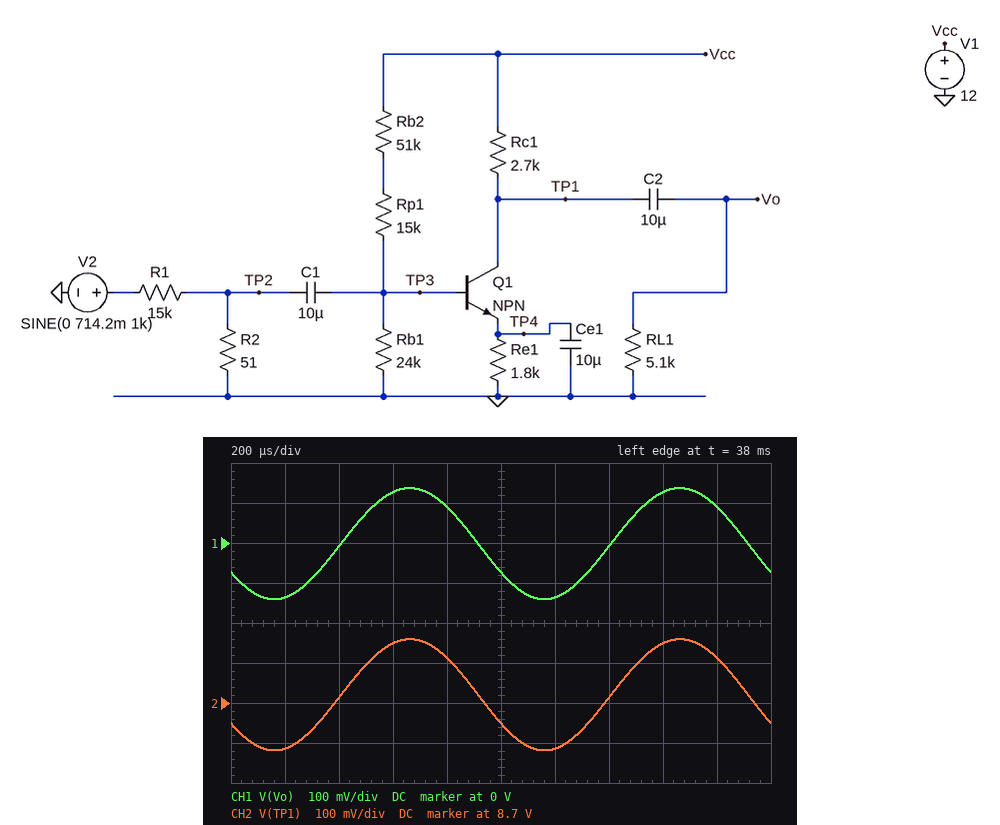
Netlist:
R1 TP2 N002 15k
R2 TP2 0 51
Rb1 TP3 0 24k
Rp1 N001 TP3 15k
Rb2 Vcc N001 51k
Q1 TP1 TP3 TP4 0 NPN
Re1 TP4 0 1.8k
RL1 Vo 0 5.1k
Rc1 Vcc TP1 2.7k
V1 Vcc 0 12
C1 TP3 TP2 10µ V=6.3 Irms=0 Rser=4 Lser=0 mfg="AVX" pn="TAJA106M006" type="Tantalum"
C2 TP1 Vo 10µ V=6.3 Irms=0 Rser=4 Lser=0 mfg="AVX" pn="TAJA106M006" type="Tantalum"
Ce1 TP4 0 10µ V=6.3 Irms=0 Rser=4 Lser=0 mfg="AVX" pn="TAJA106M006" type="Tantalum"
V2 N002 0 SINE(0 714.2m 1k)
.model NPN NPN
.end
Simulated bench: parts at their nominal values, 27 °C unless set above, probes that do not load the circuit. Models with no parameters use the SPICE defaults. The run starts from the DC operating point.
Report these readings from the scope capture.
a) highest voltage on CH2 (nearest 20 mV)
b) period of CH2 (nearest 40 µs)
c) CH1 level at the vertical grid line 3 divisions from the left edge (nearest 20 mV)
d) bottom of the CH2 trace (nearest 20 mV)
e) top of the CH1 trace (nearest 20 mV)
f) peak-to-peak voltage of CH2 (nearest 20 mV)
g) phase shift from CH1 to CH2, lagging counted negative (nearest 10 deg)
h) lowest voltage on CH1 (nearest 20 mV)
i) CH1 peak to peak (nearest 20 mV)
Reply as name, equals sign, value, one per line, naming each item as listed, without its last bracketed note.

highest voltage on CH2 = 8.86 V
period of CH2 = 1.00 ms
CH1 level at the vertical grid line 3 divisions from the left edge = 120 mV
bottom of the CH2 trace = 8.58 V
top of the CH1 trace = 140 mV
peak-to-peak voltage of CH2 = 280 mV
phase shift from CH1 to CH2, lagging counted negative = 0 deg
lowest voltage on CH1 = -140 mV
CH1 peak to peak = 280 mV
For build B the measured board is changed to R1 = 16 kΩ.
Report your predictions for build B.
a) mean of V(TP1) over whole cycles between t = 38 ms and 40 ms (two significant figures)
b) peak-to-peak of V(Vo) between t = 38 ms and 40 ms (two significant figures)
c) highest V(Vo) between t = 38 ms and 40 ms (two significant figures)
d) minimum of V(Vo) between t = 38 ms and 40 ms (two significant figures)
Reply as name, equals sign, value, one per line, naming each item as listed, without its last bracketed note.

mean of V(TP1) over whole cycles between t = 38 ms and 40 ms = 8.7 V
peak-to-peak of V(Vo) between t = 38 ms and 40 ms = 260 mV
highest V(Vo) between t = 38 ms and 40 ms = 130 mV
minimum of V(Vo) between t = 38 ms and 40 ms = -130 mV
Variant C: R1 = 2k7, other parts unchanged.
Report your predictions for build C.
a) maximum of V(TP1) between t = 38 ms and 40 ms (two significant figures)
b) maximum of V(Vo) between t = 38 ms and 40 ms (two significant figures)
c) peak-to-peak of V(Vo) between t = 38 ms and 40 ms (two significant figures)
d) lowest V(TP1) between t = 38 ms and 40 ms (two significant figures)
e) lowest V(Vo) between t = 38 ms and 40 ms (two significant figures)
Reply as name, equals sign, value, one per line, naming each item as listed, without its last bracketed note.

maximum of V(TP1) between t = 38 ms and 40 ms = 9.4 V
maximum of V(Vo) between t = 38 ms and 40 ms = 700 mV
peak-to-peak of V(Vo) between t = 38 ms and 40 ms = 1.5 V
lowest V(TP1) between t = 38 ms and 40 ms = 7.9 V
lowest V(Vo) between t = 38 ms and 40 ms = -800 mV
